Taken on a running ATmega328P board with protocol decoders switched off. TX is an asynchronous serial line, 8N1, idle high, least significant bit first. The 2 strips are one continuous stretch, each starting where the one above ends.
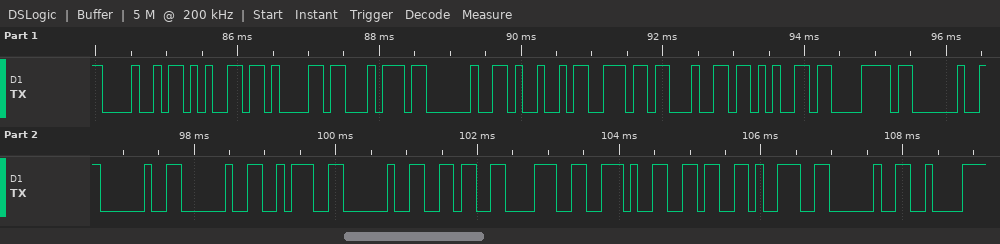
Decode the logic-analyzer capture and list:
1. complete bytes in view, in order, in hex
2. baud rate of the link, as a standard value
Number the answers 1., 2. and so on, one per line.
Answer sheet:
1. 0x48 0x65 0x61 0x74 0x20 0x49 0x6E 0x64 0x65 0x78 0x20 0x20 0x20 0x3A 0x20 0x36 0x38 0x2E 0x36 0x39 0x20 0xC2
2. 9600 baud
